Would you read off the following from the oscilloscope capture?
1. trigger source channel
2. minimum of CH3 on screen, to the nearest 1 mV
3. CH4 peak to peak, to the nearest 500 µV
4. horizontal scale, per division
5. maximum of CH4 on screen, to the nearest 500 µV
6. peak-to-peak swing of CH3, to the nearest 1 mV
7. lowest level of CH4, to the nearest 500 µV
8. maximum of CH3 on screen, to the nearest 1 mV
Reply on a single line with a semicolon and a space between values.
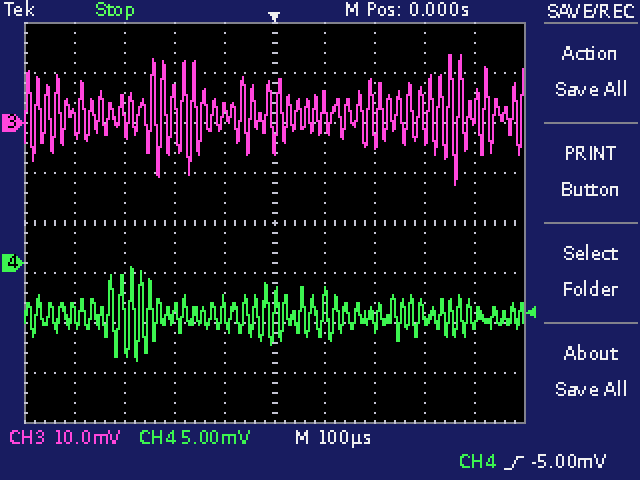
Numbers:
CH4; -12 mV; 9.5 mV; 100 µs; -500 µV; 26 mV; -10.0 mV; 14 mV
